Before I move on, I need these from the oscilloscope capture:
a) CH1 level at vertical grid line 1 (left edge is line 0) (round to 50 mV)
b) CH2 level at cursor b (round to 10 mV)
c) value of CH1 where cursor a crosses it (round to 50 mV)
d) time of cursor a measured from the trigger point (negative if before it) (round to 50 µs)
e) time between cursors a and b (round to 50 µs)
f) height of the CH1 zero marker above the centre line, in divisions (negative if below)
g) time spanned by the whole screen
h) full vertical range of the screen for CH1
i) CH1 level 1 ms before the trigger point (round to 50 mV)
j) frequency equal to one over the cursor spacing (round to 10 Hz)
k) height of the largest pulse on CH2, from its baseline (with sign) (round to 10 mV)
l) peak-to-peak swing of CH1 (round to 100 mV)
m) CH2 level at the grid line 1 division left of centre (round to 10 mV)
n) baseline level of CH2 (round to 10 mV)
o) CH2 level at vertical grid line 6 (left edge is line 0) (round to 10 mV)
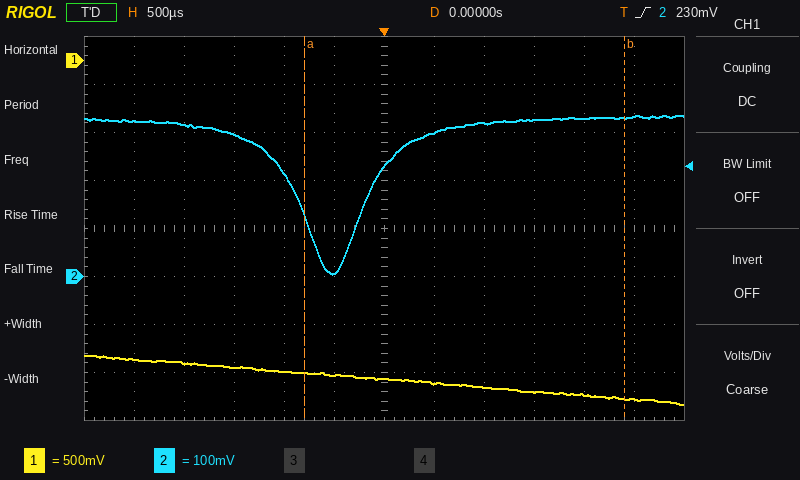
-3.10 V
330 mV
-3.25 V
-800 µs
3.20 ms
+3.5 div
6 ms
4 V
-3.25 V
310 Hz
-320 mV
500 mV
10 mV
320 mV
230 mV
